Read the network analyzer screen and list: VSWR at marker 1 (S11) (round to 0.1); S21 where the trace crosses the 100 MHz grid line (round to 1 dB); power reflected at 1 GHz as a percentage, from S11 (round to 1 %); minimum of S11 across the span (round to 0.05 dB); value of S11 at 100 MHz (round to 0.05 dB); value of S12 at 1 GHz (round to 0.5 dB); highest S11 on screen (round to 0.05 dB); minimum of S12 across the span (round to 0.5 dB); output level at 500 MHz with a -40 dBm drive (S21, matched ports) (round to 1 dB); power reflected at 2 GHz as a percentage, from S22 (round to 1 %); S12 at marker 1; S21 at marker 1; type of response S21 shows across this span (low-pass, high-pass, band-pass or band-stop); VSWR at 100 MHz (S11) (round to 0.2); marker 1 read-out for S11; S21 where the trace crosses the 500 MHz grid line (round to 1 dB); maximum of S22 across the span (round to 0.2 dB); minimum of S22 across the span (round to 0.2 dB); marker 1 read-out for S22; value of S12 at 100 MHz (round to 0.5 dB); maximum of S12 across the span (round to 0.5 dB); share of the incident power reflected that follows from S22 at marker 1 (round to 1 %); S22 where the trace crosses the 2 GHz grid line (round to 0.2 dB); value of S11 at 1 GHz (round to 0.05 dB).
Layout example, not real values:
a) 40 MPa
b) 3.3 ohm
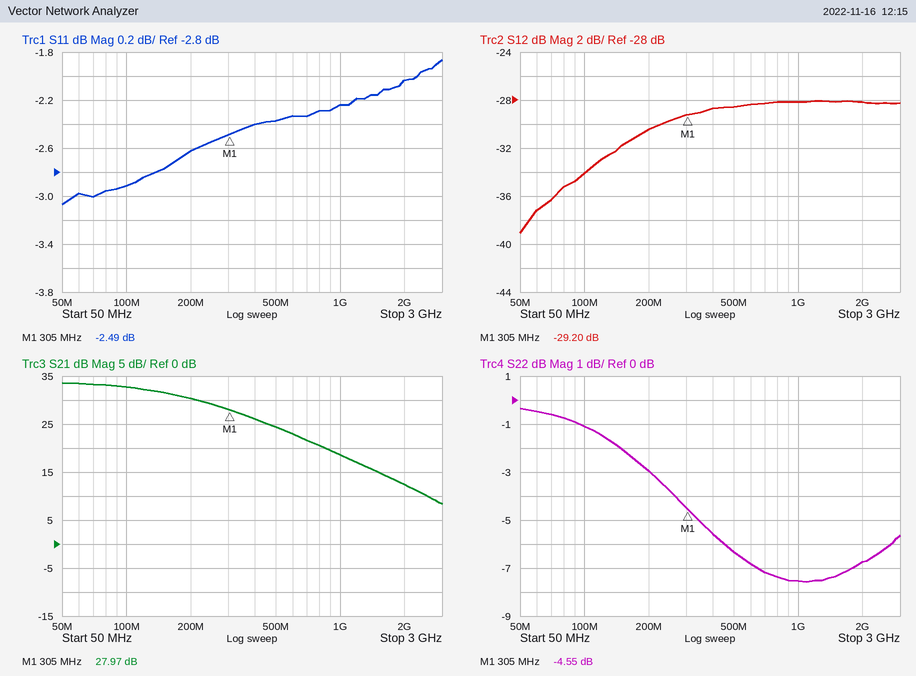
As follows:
a) 7.0
b) 33 dB
c) 60 %
d) -3.05 dB
e) -2.90 dB
f) -28.0 dB
g) -1.85 dB
h) -39.0 dB
i) -16 dBm
j) 21 %
k) -29.20 dB
l) 27.97 dB
m) low-pass
n) 6.0
o) -2.49 dB
p) 24 dB
q) -0.4 dB
r) -7.6 dB
s) -4.55 dB
t) -34.0 dB
u) -28.0 dB
v) 35 %
w) -6.8 dB
x) -2.25 dB
